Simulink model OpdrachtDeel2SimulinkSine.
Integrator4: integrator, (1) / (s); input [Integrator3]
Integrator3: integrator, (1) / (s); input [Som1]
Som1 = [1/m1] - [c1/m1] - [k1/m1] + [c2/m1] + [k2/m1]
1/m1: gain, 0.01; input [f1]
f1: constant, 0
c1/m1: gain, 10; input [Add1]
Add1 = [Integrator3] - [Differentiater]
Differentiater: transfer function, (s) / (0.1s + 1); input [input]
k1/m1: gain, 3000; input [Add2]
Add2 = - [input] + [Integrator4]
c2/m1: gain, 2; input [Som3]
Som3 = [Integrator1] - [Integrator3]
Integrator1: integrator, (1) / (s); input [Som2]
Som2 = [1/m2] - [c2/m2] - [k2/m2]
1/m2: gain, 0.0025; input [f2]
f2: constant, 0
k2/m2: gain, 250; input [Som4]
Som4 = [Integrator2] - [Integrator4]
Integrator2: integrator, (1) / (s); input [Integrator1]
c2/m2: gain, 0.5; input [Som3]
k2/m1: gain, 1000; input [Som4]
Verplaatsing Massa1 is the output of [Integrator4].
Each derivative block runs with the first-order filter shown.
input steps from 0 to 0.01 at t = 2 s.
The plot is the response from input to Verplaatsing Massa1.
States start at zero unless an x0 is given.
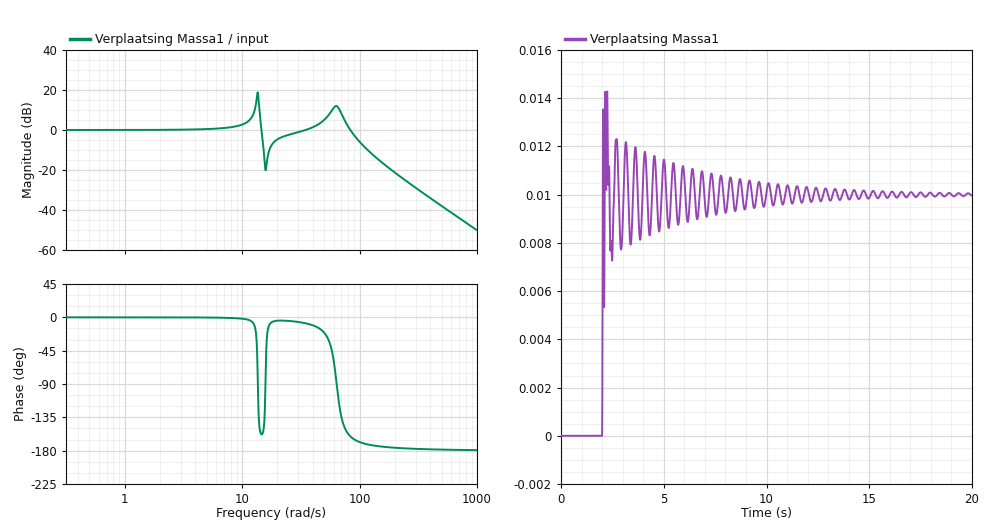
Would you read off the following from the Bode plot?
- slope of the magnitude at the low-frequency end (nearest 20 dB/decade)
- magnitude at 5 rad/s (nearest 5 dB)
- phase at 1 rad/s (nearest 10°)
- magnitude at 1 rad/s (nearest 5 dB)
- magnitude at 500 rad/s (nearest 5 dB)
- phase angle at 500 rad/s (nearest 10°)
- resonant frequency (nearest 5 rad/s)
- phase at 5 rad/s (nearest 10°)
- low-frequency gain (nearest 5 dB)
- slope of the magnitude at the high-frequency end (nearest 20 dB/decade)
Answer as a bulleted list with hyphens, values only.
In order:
- 0 dB/decade
- 0 dB
- 0°
- 0 dB
- -40 dB
- -180°
- 15 rad/s
- 0°
- 0 dB
- -40 dB/decade
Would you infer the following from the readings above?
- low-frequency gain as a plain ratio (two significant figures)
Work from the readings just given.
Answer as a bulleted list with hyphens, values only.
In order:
- 1.0
